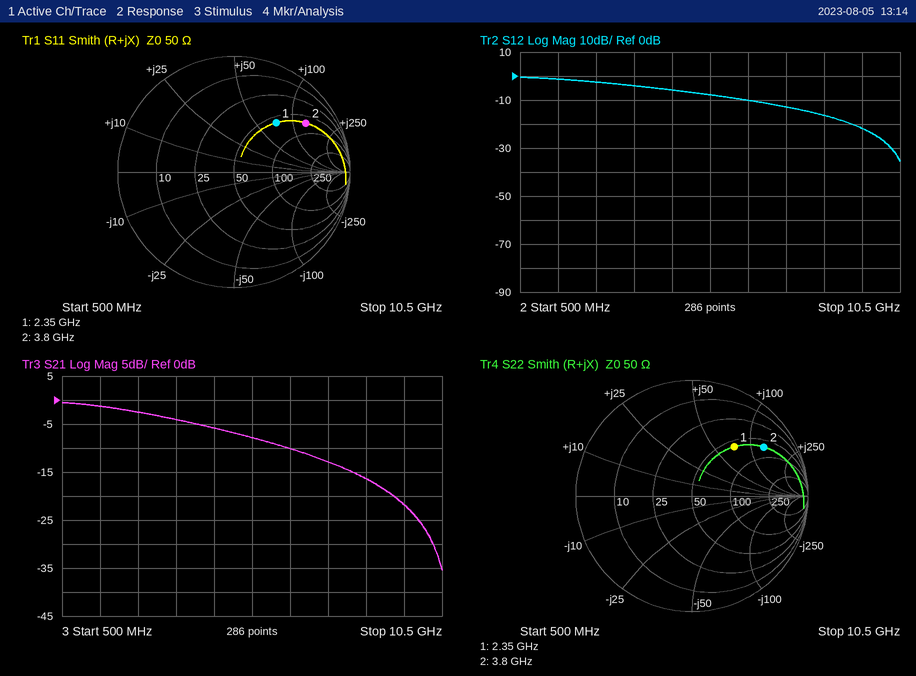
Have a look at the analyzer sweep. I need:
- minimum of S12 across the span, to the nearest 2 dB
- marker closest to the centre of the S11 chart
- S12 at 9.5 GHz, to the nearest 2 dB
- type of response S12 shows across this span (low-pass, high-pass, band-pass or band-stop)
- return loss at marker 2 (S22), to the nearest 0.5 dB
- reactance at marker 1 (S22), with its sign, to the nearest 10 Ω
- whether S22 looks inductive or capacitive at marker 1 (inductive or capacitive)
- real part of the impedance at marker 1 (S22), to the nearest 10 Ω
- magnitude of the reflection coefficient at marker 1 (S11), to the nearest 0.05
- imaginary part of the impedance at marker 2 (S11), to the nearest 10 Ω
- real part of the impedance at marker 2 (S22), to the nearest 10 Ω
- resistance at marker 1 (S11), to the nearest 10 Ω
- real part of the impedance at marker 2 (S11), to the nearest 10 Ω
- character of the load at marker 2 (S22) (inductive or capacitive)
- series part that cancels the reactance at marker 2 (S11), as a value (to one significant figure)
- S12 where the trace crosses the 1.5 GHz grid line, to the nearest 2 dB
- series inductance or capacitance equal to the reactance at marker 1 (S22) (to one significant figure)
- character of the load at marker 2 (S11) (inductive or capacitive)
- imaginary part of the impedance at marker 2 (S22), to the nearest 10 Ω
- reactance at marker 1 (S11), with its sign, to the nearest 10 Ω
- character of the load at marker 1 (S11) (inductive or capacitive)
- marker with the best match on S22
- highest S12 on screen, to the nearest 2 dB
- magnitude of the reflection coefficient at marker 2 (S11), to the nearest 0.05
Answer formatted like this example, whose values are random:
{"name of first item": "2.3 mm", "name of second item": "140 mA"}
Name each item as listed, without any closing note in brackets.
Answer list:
{"minimum of S12 across the span, to the nearest 2 dB": "-36 dB", "marker closest to the centre of the S11 chart": "marker 1", "S12 at 9.5 GHz, to the nearest 2 dB": "-22 dB", "type of response S12 shows across this span": "low-pass", "return loss at marker 2 (S22), to the nearest 0.5 dB": "2.5 dB", "reactance at marker 1 (S22), with its sign, to the nearest 10 Ω": "+70 Ω", "whether S22 looks inductive or capacitive at marker 1": "inductive", "real part of the impedance at marker 1 (S22), to the nearest 10 Ω": "60 Ω", "magnitude of the reflection coefficient at marker 1 (S11), to the nearest 0.05": "0.55", "imaginary part of the impedance at marker 2 (S11), to the nearest 10 Ω": "+130 Ω", "real part of the impedance at marker 2 (S22), to the nearest 10 Ω": "70 Ω", "resistance at marker 1 (S11), to the nearest 10 Ω": "60 Ω", "real part of the impedance at marker 2 (S11), to the nearest 10 Ω": "70 Ω", "character of the load at marker 2 (S22)": "inductive", "series part that cancels the reactance at marker 2 (S11), as a value": "300 fF", "S12 where the trace crosses the 1.5 GHz grid line, to the nearest 2 dB": "-2 dB", "series inductance or capacitance equal to the reactance at marker 1 (S22)": "5 nH", "character of the load at marker 2 (S11)": "inductive", "imaginary part of the impedance at marker 2 (S22), to the nearest 10 Ω": "+130 Ω", "reactance at marker 1 (S11), with its sign, to the nearest 10 Ω": "+70 Ω", "character of the load at marker 1 (S11)": "inductive", "marker with the best match on S22": "marker 1", "highest S12 on screen, to the nearest 2 dB": "0 dB", "magnitude of the reflection coefficient at marker 2 (S11), to the nearest 0.05": "0.75"}
